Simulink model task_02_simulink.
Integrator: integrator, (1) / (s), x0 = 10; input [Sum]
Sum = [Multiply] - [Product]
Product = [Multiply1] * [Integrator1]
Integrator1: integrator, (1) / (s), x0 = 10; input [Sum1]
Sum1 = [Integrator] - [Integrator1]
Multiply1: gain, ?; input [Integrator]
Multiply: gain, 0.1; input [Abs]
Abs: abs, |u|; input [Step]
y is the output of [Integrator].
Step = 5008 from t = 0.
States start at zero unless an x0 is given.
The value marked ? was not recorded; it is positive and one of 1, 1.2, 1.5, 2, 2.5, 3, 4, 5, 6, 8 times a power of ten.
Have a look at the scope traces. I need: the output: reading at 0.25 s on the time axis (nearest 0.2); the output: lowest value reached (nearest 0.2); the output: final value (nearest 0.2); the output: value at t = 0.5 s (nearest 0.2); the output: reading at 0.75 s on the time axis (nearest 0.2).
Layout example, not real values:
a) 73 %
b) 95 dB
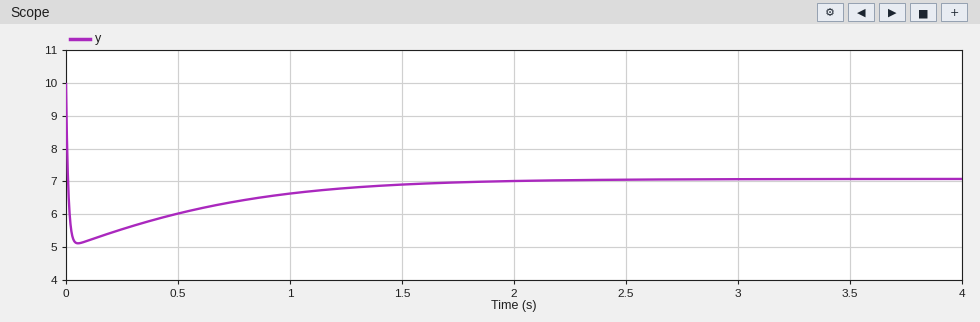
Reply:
a) 5.6
b) 5.2
c) 7.0
d) 6.0
e) 6.4
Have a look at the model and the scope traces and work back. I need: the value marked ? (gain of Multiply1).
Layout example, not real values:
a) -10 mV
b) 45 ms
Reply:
a) 10
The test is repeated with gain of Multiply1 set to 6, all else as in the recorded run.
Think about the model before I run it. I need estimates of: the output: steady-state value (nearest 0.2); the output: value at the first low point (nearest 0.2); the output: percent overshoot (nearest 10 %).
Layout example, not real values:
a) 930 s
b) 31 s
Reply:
a) 9.2
b) 8.4
c) 80 %
